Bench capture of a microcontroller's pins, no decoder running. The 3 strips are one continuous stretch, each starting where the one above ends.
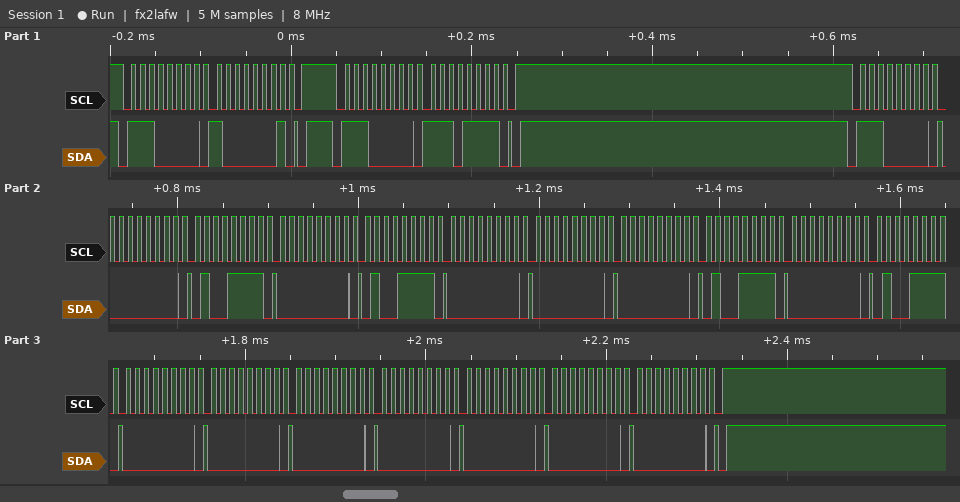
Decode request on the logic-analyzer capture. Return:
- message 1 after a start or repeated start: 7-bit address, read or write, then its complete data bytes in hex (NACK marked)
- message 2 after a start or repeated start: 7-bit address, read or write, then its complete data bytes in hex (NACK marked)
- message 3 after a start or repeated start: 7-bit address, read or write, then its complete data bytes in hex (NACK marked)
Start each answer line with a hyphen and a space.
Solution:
- 0x70 write: 81
- 0x70 write: EF
- 0x70 write: 00 4F 00 4F 00 00 00 4F 00 4F 00 00 00 00 00 00 00
